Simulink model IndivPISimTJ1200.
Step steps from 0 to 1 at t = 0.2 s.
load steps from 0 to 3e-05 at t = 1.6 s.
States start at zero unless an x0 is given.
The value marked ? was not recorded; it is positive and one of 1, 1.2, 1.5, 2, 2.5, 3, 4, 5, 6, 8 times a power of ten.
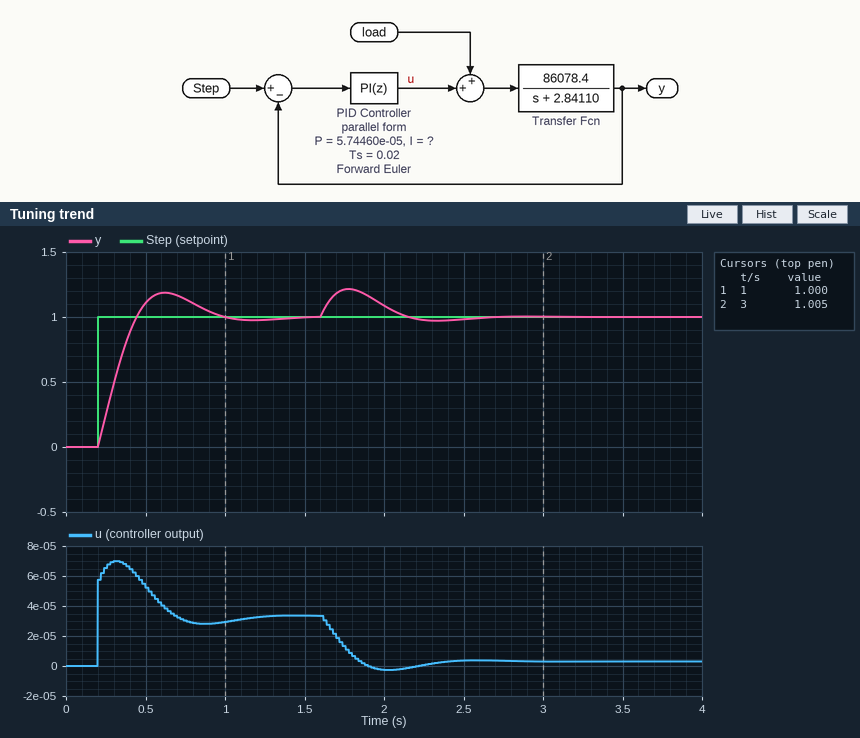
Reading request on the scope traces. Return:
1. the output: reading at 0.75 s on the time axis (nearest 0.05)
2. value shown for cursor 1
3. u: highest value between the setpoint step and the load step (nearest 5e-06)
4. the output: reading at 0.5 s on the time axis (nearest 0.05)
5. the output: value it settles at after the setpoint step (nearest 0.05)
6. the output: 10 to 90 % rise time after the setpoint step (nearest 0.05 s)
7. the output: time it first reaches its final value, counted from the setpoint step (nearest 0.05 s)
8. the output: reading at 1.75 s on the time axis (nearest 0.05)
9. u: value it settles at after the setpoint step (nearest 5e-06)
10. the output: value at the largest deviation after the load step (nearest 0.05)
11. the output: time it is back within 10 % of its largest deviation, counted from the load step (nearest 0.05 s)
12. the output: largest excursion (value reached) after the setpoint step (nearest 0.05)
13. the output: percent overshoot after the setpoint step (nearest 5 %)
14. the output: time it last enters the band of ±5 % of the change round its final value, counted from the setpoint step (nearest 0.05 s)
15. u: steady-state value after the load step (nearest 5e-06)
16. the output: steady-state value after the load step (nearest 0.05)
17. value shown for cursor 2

1.15
1.000
0.000070
1.10
1.00
0.20 s
0.25 s
1.20
0.000035
1.20
0.85 s
1.20
20 %
0.70 s
0.000005
1.00
1.005
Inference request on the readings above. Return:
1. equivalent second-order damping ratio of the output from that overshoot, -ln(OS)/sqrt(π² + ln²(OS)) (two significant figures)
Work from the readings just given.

0.46
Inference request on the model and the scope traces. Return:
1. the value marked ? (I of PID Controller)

0.0005
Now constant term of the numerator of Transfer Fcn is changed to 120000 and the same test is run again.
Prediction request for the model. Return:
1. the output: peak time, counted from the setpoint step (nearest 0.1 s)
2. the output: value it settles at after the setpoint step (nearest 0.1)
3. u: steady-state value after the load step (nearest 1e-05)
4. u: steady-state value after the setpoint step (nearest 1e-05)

0.3 s
1.0
-0.00001
0.00002
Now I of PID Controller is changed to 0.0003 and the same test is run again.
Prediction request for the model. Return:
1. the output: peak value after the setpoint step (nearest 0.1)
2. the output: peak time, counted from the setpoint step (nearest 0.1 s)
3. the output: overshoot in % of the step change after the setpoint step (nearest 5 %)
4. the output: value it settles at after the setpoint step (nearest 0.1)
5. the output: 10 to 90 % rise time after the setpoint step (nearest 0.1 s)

1.1
0.6 s
10 %
1.0
0.3 s
